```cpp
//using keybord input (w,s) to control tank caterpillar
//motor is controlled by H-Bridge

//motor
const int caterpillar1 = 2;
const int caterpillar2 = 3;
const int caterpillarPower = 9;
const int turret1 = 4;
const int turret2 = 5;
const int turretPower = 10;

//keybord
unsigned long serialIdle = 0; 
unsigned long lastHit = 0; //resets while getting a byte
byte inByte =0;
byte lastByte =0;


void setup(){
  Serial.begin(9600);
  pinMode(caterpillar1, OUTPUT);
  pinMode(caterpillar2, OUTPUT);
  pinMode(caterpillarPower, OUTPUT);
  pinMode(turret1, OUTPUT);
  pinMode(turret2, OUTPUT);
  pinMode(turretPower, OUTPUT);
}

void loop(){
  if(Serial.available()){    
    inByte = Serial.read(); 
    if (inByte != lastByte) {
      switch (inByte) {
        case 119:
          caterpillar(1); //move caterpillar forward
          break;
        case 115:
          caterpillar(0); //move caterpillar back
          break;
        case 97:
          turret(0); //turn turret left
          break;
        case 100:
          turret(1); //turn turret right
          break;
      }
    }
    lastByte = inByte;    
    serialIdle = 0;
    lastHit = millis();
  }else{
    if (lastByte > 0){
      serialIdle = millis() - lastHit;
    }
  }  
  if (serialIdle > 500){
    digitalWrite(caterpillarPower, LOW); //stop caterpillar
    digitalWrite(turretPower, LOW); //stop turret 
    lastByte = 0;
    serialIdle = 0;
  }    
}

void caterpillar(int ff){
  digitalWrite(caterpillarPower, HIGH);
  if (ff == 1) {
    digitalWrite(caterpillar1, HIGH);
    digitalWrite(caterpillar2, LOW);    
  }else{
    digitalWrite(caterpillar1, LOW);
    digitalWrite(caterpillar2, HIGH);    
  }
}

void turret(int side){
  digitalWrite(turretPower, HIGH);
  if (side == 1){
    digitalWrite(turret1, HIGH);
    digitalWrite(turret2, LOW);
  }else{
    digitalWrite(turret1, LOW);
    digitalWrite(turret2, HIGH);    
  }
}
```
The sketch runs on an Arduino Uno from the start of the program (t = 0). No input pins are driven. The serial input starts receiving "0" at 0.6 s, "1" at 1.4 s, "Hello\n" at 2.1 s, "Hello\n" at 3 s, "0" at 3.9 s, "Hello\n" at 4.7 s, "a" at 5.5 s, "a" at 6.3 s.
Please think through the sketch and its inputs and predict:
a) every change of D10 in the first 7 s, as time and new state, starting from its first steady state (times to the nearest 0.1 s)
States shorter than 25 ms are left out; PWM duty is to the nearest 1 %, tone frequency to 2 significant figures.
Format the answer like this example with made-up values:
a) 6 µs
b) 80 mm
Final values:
a) 0 s low; 5.5 s high; 6 s low; 6.3 s high; 6.8 s low
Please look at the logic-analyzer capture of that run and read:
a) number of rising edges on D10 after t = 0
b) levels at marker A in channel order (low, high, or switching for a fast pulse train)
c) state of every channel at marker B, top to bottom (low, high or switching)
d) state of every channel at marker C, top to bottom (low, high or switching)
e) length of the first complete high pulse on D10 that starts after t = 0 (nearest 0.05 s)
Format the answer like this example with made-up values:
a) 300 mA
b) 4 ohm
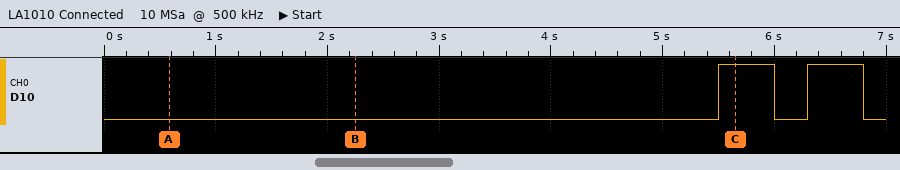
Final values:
a) 2
b) D10 low
c) D10 low
d) D10 high
e) 0.50 s
